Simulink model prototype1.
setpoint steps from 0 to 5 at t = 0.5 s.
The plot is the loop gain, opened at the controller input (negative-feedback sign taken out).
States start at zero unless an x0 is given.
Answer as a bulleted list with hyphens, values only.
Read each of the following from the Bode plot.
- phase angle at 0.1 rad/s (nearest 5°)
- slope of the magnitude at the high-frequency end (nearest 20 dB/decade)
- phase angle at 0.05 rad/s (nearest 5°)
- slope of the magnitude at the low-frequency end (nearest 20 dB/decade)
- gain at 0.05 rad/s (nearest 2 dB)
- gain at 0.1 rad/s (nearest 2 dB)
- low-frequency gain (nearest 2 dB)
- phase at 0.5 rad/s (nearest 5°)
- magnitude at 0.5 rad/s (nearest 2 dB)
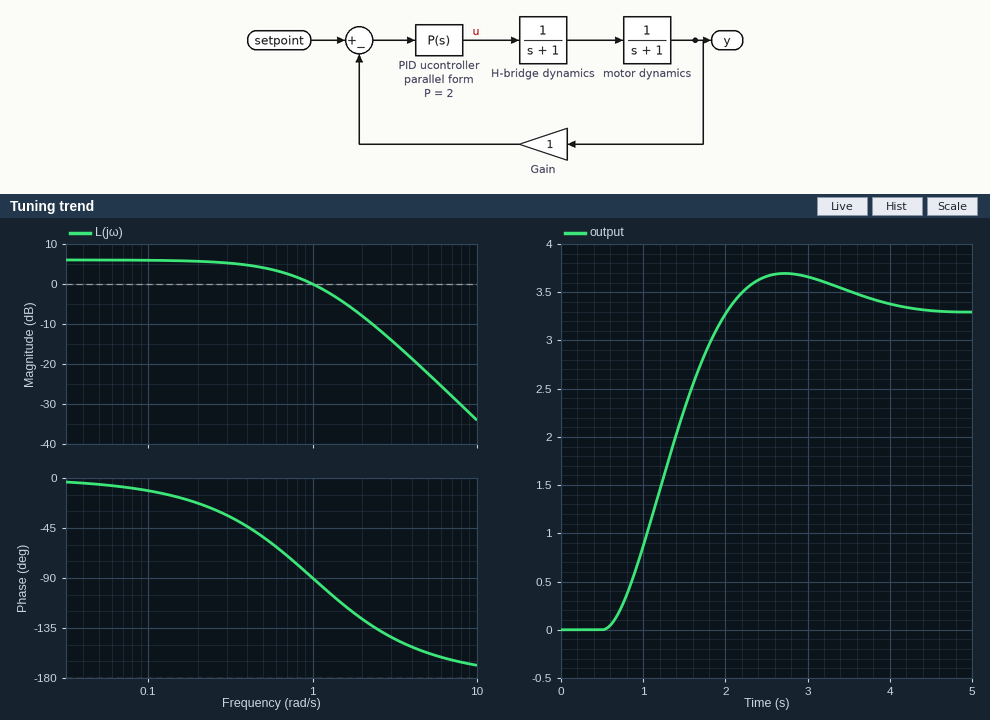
- -10°
- -40 dB/decade
- -5°
- 0 dB/decade
- 6 dB
- 6 dB
- 6 dB
- -55°
- 4 dB
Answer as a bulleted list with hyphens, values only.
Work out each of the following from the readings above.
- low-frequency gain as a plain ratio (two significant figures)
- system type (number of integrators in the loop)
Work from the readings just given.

- 2.0
- 0
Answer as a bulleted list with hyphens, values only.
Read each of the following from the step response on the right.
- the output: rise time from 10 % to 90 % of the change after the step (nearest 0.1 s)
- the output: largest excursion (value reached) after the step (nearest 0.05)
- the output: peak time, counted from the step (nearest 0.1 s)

- 1.0 s
- 3.70
- 2.2 s
